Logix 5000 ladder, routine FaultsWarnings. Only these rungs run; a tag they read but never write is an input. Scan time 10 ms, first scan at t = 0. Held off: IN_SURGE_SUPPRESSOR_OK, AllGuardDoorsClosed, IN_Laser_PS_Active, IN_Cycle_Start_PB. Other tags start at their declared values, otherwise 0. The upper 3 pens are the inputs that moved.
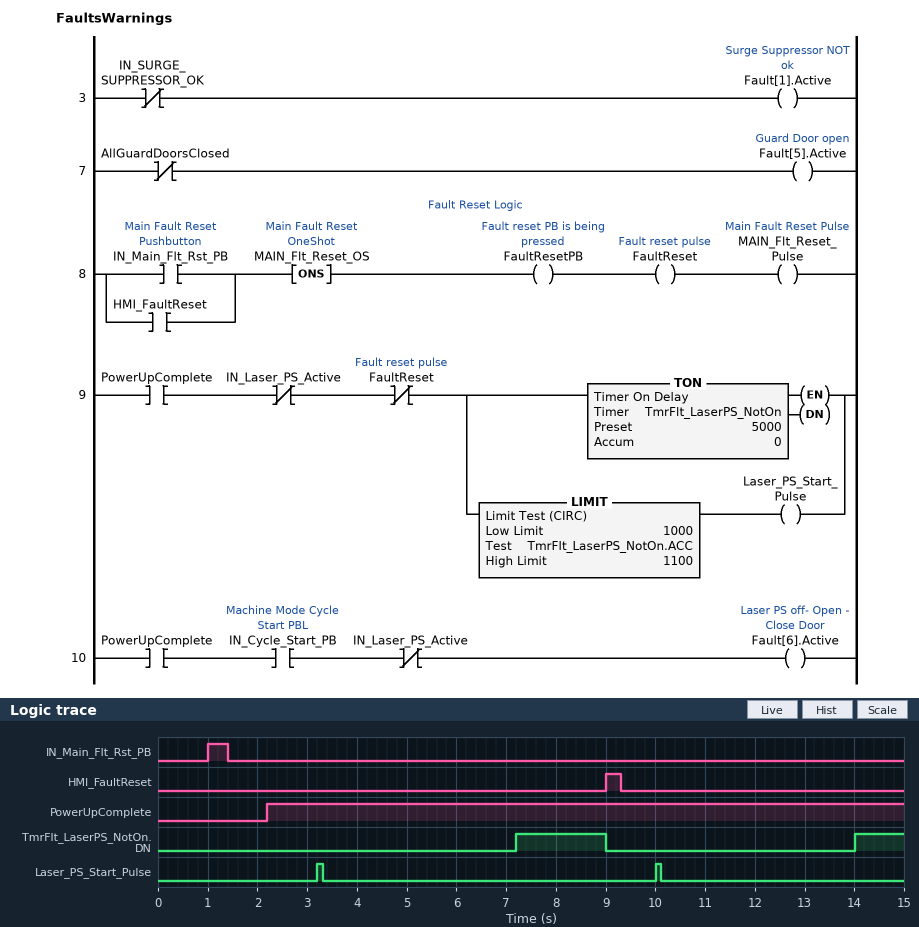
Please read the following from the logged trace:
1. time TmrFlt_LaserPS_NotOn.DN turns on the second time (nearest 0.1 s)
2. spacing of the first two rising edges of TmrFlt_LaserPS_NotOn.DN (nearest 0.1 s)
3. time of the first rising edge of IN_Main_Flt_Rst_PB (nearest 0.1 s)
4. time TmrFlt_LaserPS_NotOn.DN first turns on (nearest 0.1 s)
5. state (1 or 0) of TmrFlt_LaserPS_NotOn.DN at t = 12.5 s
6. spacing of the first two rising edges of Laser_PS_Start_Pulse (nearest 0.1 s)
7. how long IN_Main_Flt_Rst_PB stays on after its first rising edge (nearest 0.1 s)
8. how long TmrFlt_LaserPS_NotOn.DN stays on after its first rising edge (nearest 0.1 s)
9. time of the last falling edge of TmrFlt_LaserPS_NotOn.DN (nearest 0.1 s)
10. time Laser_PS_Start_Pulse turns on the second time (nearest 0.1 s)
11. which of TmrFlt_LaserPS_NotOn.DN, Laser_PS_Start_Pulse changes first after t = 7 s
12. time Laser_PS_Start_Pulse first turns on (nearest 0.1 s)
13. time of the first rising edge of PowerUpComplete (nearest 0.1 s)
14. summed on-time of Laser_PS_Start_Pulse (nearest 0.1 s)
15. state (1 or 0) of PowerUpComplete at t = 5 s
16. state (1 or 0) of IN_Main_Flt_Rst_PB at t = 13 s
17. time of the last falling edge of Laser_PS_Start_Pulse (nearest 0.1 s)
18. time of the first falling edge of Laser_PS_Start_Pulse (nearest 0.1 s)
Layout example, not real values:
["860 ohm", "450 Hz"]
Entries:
["14.0 s", "6.8 s", "1.0 s", "7.2 s", "0", "6.8 s", "0.4 s", "1.8 s", "9.0 s", "10.0 s", "TmrFlt_LaserPS_NotOn.DN", "3.2 s", "2.2 s", "0.2 s", "1", "0", "10.1 s", "3.3 s"]
